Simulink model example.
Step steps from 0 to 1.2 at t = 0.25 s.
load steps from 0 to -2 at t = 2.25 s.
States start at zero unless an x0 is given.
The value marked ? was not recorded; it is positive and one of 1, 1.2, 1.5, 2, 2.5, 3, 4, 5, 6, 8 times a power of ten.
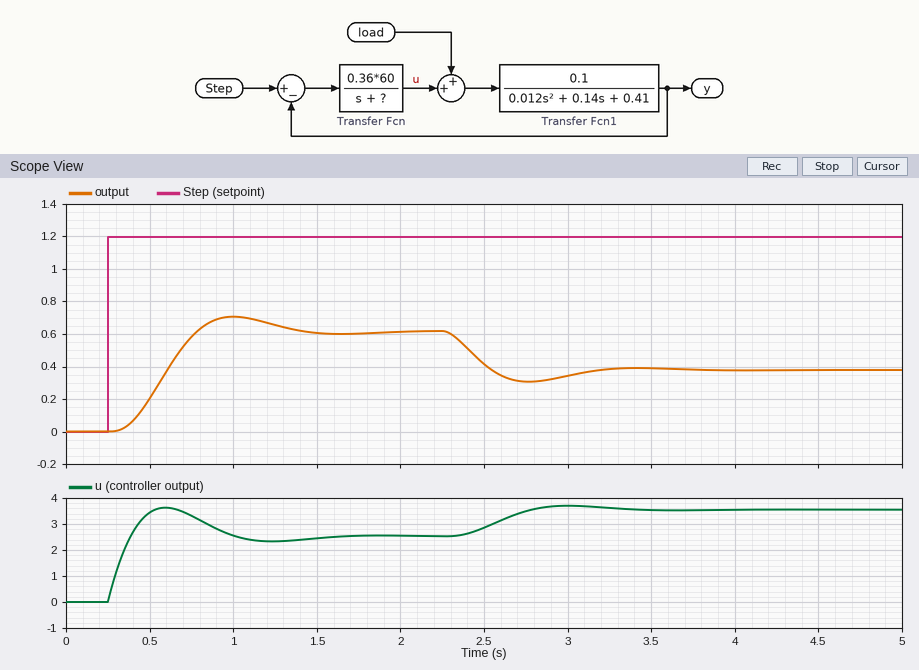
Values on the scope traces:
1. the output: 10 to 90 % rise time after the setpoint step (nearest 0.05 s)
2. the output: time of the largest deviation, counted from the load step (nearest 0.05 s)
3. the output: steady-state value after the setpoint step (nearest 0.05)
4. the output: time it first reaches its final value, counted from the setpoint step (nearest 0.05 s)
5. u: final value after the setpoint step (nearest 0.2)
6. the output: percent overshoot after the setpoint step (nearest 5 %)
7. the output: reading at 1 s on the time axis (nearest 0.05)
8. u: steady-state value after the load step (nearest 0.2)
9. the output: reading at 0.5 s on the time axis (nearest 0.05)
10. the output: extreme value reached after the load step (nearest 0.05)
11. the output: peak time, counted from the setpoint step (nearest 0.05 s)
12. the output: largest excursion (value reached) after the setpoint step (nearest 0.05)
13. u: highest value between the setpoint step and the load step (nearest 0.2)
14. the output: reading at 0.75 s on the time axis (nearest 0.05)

0.35 s
0.50 s
0.60
0.55 s
2.6
15 %
0.70
3.6
0.20
0.30
0.75 s
0.70
3.6
0.60
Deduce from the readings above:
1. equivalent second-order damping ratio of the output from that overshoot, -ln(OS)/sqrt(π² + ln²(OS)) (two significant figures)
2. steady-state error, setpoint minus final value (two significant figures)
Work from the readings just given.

0.52
0.60
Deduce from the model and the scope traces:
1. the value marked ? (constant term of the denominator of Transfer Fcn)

5
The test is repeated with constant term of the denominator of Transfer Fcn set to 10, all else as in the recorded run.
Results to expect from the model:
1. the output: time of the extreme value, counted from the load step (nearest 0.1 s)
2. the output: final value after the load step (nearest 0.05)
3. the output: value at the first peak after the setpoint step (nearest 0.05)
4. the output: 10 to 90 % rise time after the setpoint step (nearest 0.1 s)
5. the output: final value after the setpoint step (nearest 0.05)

0.6 s
0.10
0.45
0.4 s
0.40
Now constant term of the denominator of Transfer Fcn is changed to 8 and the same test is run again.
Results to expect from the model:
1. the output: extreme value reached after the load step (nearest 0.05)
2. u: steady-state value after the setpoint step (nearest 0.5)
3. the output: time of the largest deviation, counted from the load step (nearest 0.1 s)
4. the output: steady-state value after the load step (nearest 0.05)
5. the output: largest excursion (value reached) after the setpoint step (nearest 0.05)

0.15
2.0
0.6 s
0.20
0.50
